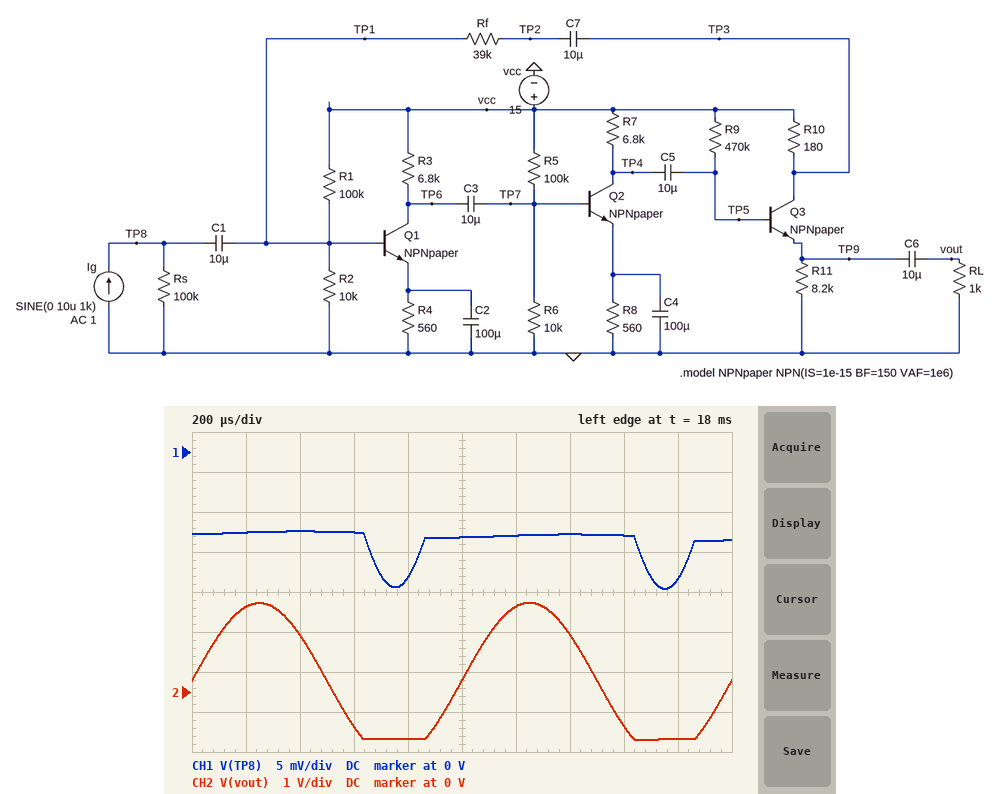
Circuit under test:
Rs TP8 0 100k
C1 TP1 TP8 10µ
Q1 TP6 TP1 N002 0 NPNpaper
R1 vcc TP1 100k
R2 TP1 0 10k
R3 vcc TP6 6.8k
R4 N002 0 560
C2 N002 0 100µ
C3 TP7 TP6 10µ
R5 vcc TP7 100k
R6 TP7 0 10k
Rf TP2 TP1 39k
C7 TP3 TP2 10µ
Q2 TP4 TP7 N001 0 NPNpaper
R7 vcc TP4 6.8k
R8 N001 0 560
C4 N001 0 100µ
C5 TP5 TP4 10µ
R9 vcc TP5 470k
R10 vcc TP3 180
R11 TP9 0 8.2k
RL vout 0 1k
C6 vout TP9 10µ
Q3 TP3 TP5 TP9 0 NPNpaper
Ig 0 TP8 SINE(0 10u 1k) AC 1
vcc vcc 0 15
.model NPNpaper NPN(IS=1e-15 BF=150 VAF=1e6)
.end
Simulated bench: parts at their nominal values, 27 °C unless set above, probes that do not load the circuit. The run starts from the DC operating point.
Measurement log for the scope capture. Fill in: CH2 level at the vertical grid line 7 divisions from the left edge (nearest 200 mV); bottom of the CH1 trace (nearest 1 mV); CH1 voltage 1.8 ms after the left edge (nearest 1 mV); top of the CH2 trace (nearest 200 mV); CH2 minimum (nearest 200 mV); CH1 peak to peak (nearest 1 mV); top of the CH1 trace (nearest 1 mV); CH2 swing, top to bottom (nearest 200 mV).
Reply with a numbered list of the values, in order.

1. 1.4 V
2. -17 mV
3. -16 mV
4. 2.2 V
5. -1.2 V
6. 7 mV
7. -10 mV
8. 3.4 V
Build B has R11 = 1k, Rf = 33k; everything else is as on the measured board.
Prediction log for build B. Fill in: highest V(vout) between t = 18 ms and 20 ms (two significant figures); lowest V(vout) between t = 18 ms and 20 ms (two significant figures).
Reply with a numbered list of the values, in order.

1. 920 mV
2. -930 mV
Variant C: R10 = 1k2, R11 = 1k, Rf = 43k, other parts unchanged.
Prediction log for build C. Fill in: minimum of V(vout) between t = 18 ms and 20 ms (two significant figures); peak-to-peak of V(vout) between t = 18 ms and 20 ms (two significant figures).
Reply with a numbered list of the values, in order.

1. -190 mV
2. 370 mV
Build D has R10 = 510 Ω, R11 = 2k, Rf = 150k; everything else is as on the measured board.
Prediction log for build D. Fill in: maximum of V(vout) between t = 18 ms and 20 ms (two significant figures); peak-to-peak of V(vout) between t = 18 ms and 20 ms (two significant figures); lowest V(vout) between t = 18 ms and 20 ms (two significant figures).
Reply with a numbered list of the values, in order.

1. 2.0 V
2. 3.9 V
3. -1.9 V
